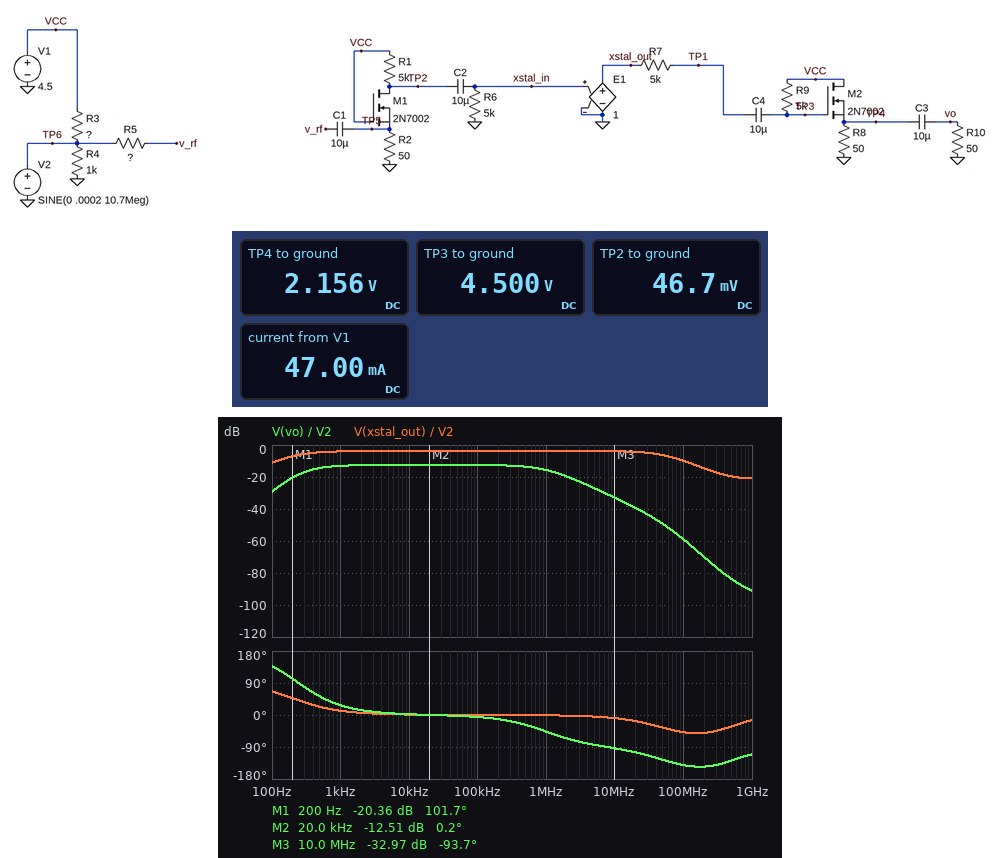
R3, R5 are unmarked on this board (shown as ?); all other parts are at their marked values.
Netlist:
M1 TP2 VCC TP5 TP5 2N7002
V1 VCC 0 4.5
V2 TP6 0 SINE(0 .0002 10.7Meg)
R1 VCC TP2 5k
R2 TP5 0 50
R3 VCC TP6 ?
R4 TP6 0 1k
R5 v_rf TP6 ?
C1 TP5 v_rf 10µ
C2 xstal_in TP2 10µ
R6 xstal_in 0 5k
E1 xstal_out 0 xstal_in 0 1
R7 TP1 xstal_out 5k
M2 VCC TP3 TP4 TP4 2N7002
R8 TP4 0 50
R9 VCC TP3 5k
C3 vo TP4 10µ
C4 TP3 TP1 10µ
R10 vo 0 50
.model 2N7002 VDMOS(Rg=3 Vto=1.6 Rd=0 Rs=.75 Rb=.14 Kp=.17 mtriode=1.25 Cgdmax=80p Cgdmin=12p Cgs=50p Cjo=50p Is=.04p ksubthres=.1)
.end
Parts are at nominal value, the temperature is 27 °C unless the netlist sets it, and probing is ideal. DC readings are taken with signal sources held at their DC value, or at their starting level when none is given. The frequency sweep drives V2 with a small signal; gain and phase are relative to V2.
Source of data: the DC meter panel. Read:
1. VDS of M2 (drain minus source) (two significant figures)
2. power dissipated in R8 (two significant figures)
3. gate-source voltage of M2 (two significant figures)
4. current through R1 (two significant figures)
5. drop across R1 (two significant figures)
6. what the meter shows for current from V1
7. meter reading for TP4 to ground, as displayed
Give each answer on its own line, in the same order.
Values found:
2.3 V
93 mW
2.3 V
890 µA
4.5 V
47.00 mA
2.156 V
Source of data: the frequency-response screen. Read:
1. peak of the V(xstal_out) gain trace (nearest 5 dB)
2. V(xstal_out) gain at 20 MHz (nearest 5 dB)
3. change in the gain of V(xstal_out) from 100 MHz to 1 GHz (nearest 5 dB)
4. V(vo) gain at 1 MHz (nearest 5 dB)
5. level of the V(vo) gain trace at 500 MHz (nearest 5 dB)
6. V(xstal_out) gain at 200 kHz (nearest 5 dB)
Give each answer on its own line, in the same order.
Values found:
-5 dB
-5 dB
-10 dB
-15 dB
-85 dB
-5 dB
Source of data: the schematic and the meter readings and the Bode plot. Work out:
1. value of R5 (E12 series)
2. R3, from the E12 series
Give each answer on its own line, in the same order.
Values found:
27 Ω
1.5 kΩ
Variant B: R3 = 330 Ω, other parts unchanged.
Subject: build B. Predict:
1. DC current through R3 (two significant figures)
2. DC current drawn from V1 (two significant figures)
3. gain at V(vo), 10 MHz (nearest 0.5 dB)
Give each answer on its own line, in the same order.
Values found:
14 mA
58 mA
-33.0 dB
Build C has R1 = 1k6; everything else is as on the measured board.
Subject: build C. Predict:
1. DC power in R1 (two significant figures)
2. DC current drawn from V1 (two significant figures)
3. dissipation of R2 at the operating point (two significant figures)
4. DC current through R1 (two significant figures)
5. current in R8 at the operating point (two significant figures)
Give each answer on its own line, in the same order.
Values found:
12 mW
49 mA
370 µW
2.7 mA
43 mA
